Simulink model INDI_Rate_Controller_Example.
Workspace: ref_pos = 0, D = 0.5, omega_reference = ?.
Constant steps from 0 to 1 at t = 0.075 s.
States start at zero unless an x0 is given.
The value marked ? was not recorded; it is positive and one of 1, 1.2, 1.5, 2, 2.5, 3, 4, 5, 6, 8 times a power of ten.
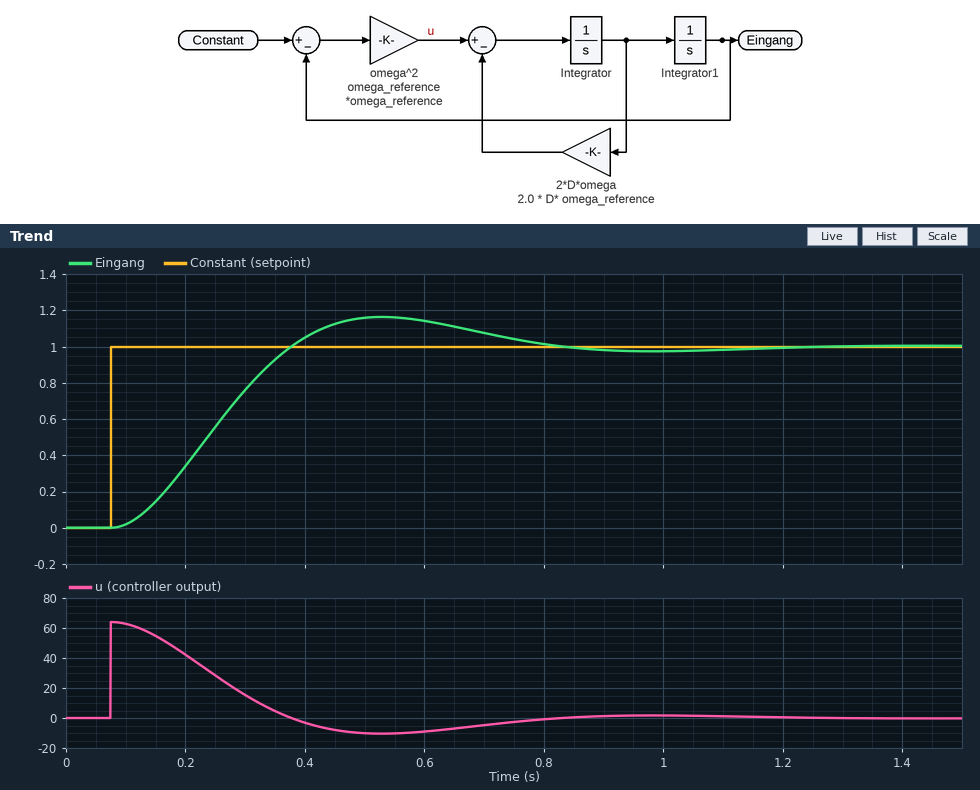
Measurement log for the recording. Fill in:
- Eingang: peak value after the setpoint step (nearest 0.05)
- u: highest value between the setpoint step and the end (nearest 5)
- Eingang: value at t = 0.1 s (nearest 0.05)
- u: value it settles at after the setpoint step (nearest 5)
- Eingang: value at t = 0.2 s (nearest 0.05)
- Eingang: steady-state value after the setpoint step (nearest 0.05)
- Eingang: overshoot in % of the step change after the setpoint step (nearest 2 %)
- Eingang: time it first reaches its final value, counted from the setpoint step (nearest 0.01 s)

1.15
65
0.00
0
0.35
1.00
16 %
0.30 s
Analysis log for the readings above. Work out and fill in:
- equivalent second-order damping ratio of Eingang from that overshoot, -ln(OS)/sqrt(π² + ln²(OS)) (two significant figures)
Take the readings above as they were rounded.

0.50
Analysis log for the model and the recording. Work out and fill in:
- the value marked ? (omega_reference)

8
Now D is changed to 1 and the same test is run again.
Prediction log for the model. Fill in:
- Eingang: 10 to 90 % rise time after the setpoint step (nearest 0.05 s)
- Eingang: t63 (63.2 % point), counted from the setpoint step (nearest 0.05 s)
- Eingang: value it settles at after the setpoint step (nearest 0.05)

0.40 s
0.25 s
1.00
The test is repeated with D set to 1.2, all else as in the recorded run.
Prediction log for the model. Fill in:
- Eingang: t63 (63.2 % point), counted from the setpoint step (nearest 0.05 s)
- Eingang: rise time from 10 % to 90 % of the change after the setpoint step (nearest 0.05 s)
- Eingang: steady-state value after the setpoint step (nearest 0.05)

0.30 s
0.55 s
1.00
